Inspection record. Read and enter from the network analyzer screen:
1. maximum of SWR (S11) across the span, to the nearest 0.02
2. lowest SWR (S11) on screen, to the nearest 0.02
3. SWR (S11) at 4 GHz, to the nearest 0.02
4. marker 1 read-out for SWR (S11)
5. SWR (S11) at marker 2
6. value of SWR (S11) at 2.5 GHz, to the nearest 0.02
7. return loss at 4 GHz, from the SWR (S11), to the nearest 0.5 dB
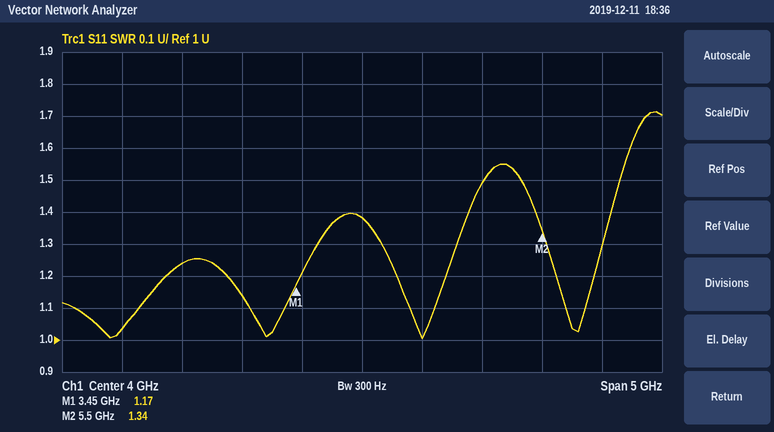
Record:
1.72
1.00
1.38
1.17
1.34
1.24
16.0 dB
